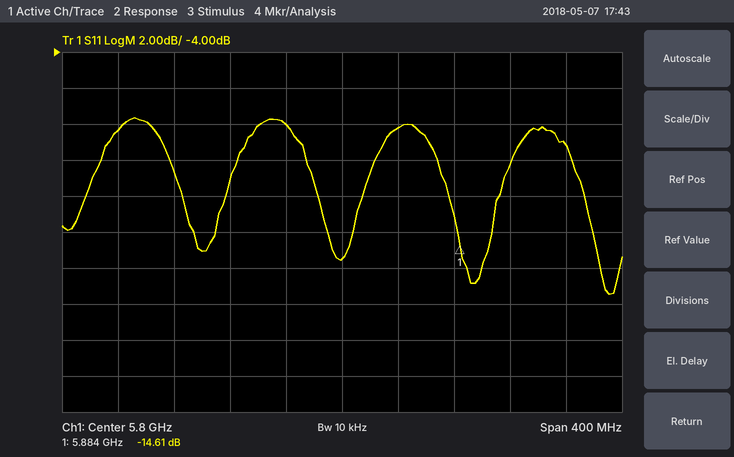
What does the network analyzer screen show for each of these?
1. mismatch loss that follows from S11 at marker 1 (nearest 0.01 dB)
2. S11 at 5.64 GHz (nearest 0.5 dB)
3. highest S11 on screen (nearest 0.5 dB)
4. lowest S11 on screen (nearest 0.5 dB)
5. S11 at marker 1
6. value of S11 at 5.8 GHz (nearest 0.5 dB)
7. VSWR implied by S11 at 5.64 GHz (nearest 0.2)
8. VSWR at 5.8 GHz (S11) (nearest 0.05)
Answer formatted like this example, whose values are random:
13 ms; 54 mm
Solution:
0.15 dB; -8.5 dB; -7.5 dB; -17.5 dB; -14.61 dB; -15.5 dB; 2.2; 1.40
